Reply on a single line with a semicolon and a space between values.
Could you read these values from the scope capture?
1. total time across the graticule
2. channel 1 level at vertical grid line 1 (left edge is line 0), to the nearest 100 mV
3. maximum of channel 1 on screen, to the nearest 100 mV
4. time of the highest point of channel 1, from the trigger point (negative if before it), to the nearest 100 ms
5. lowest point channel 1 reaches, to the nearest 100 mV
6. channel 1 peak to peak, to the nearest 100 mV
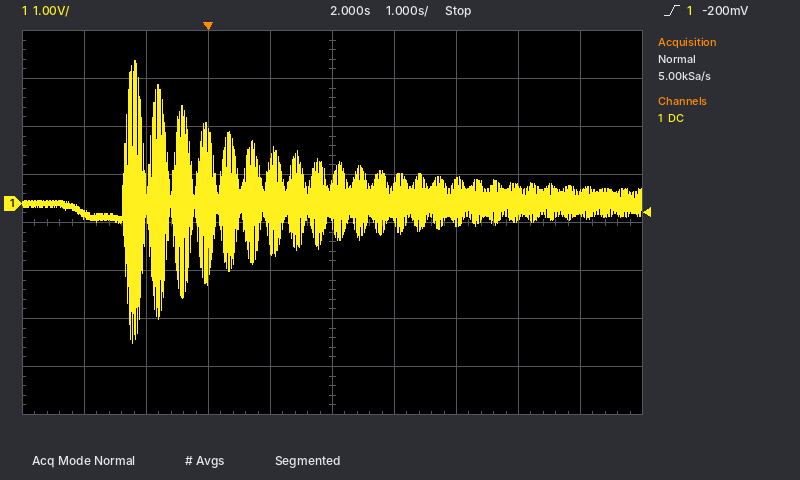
10 s; -200 mV; 3.0 V; -1.2 s; -2.9 V; 5.9 V
